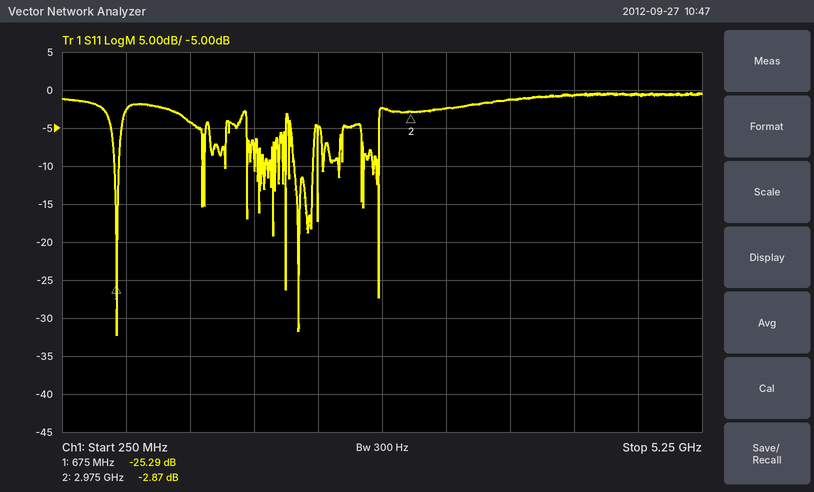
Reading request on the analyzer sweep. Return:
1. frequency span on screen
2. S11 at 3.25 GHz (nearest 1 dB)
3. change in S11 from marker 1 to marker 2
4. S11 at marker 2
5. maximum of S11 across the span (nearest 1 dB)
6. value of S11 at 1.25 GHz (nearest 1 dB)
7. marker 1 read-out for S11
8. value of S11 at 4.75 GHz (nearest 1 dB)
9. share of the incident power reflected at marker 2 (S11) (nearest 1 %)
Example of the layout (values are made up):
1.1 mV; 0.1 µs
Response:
5 GHz; -2 dB; 22.42 dB; -2.87 dB; 0 dB; -4 dB; -25.29 dB; -1 dB; 52 %
